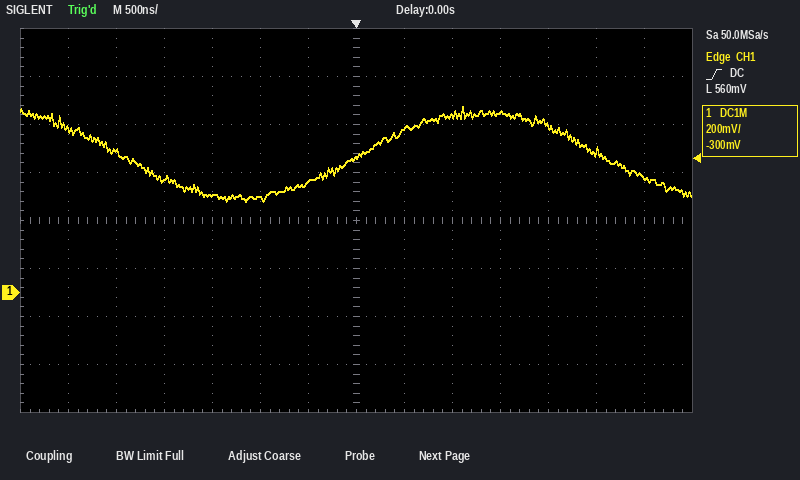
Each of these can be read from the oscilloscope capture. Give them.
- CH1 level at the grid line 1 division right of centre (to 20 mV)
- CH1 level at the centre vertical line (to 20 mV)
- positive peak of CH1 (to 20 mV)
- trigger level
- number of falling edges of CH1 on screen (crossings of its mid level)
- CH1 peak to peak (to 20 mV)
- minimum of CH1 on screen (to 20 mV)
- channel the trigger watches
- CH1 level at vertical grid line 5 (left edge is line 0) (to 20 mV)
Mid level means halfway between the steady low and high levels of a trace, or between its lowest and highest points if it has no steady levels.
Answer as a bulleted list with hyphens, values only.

- 680 mV
- 560 mV
- 780 mV
- 560 mV
- 2
- 400 mV
- 380 mV
- CH1
- 400 mV
